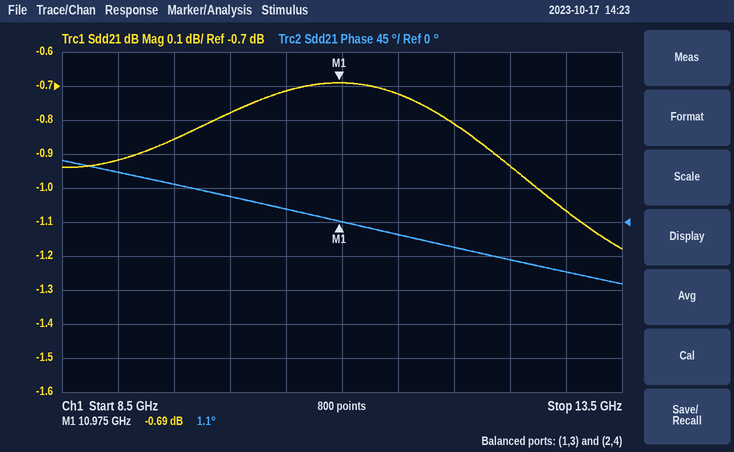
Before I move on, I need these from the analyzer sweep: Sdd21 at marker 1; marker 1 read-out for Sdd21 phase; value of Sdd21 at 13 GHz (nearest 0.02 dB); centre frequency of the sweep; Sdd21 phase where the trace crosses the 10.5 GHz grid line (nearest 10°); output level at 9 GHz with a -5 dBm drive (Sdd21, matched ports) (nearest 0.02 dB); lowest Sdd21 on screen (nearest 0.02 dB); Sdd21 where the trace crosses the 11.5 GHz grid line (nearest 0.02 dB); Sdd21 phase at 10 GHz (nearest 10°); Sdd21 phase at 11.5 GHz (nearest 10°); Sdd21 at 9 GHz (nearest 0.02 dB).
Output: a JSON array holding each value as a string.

["-0.69 dB", "1.1°", "-1.06 dB", "11 GHz", "20°", "-5.92 dBm", "-1.18 dB", "-0.72 dB", "30°", "-20°", "-0.92 dB"]
